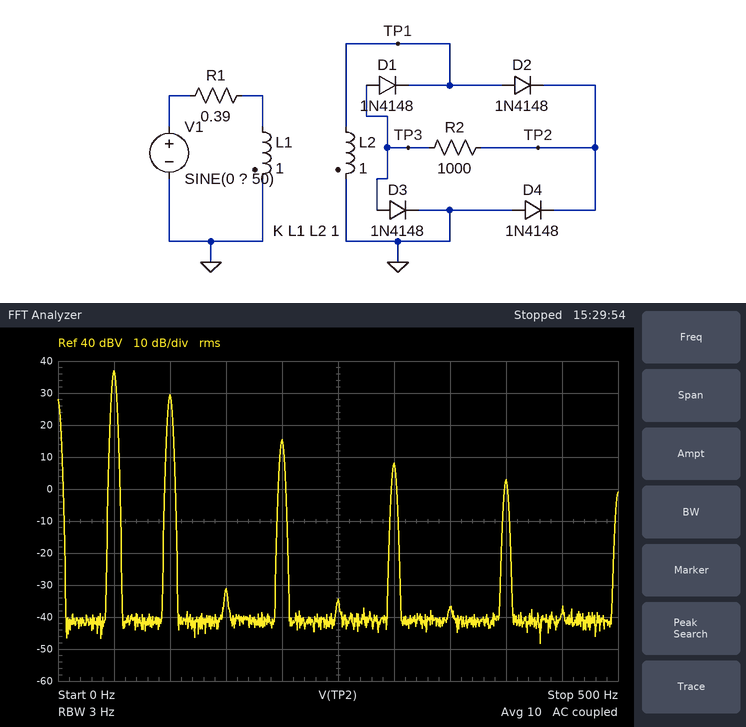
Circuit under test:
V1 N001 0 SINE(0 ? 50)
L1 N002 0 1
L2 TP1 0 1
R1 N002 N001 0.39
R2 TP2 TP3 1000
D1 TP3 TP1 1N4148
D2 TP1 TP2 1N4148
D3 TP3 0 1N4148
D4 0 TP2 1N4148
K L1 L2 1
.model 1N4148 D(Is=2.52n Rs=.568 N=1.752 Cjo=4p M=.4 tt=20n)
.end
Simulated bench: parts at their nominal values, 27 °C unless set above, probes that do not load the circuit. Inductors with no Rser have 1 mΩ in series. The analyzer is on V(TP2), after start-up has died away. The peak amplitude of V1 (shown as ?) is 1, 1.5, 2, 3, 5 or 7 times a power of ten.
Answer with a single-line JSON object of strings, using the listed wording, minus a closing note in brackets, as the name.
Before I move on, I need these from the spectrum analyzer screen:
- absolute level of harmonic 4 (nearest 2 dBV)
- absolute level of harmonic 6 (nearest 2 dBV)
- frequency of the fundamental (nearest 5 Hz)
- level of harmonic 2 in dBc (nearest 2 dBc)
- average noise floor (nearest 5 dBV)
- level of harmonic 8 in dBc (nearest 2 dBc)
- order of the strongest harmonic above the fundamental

{"absolute level of harmonic 4": "16 dBV", "absolute level of harmonic 6": "8 dBV", "frequency of the fundamental": "50 Hz", "level of harmonic 2 in dBc": "-8 dBc", "average noise floor": "-40 dBV", "level of harmonic 8 in dBc": "-34 dBc", "order of the strongest harmonic above the fundamental": "2"}
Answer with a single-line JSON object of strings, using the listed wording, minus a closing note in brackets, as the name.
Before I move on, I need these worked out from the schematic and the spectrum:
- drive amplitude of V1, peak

{"drive amplitude of V1, peak": "200 V"}
